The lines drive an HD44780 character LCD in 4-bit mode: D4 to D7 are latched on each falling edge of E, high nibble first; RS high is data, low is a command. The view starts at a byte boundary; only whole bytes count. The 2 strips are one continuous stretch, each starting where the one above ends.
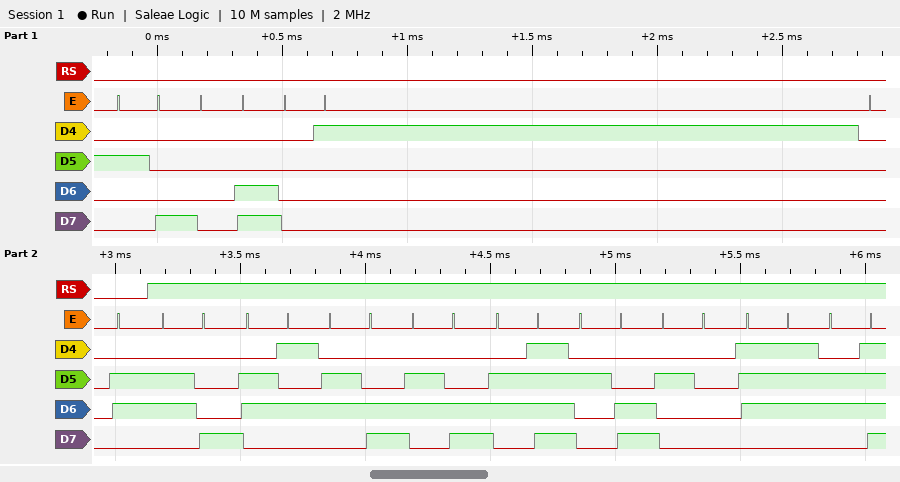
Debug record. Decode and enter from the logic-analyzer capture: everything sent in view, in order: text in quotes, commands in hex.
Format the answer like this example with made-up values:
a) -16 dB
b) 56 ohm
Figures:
a) 0x28 0x0C 0x01 0x06 "hello, wo"
